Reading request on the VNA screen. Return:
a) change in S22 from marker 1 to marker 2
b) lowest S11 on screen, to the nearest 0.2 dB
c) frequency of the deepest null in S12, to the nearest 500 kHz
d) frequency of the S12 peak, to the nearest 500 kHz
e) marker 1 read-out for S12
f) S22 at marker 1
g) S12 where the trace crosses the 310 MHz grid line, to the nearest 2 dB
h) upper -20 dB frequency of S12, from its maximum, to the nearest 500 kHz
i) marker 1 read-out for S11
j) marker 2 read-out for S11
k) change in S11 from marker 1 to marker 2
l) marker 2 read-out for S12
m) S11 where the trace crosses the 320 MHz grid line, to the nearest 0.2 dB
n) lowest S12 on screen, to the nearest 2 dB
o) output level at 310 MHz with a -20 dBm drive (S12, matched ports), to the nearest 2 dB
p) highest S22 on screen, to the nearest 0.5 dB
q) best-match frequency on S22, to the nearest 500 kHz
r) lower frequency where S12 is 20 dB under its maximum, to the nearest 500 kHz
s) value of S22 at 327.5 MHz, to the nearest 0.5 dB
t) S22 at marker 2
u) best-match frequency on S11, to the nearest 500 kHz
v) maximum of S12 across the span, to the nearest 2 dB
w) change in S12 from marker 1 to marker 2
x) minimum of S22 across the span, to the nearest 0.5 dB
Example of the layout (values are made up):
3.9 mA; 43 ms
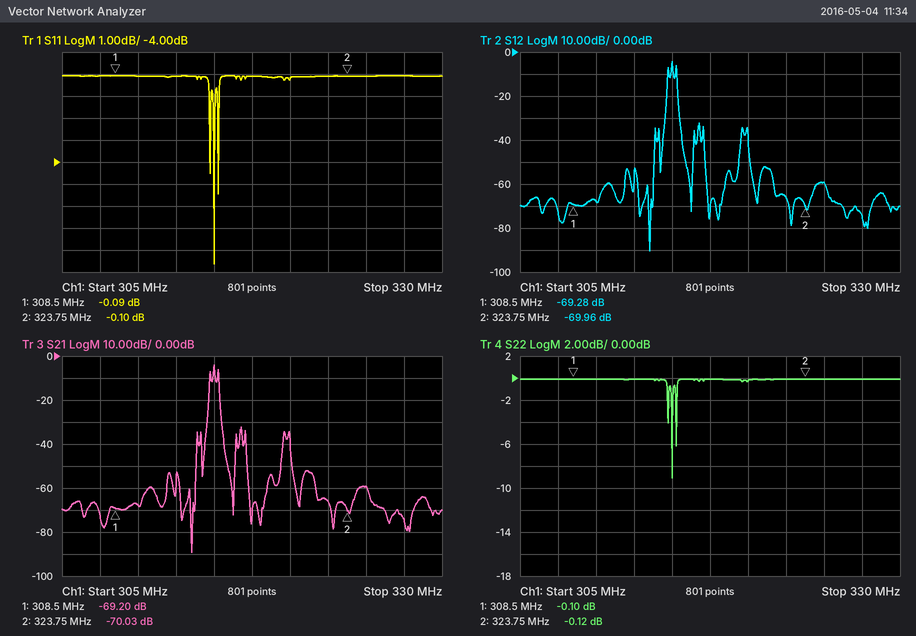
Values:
-0.02 dB; -8.6 dB; 313.5 MHz; 315.0 MHz; -69.28 dB; -0.10 dB; -68 dB; 315.5 MHz; -0.09 dB; -0.10 dB; -0.01 dB; -69.96 dB; -0.2 dB; -90 dB; -88 dBm; 0.0 dB; 315.0 MHz; 314.5 MHz; 0.0 dB; -0.12 dB; 315.0 MHz; -4 dB; -0.68 dB; -9.0 dB
